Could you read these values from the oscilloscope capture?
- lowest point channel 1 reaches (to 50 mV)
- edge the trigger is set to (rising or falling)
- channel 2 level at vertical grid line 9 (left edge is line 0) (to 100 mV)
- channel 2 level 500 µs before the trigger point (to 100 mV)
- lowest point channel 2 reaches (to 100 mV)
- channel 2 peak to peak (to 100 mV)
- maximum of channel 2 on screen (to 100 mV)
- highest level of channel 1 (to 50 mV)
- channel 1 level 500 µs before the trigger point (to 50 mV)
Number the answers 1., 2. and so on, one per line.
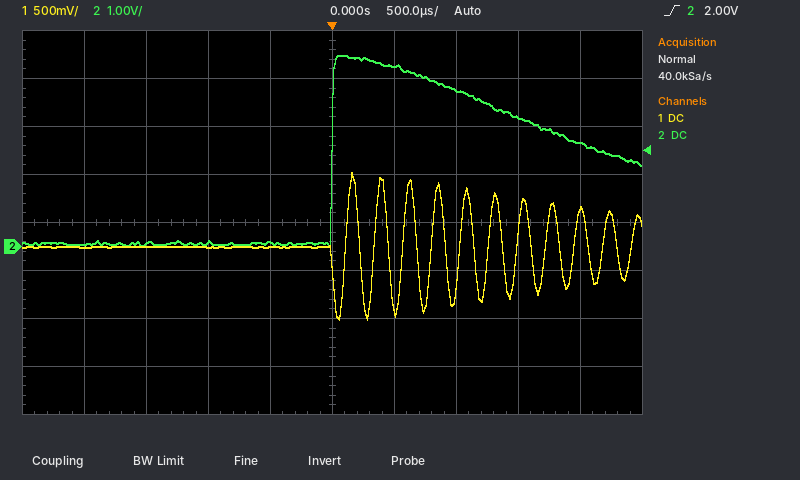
1. -750 mV
2. rising
3. 2.2 V
4. 100 mV
5. 0.0 V
6. 4.0 V
7. 4.0 V
8. 750 mV
9. 0 mV
